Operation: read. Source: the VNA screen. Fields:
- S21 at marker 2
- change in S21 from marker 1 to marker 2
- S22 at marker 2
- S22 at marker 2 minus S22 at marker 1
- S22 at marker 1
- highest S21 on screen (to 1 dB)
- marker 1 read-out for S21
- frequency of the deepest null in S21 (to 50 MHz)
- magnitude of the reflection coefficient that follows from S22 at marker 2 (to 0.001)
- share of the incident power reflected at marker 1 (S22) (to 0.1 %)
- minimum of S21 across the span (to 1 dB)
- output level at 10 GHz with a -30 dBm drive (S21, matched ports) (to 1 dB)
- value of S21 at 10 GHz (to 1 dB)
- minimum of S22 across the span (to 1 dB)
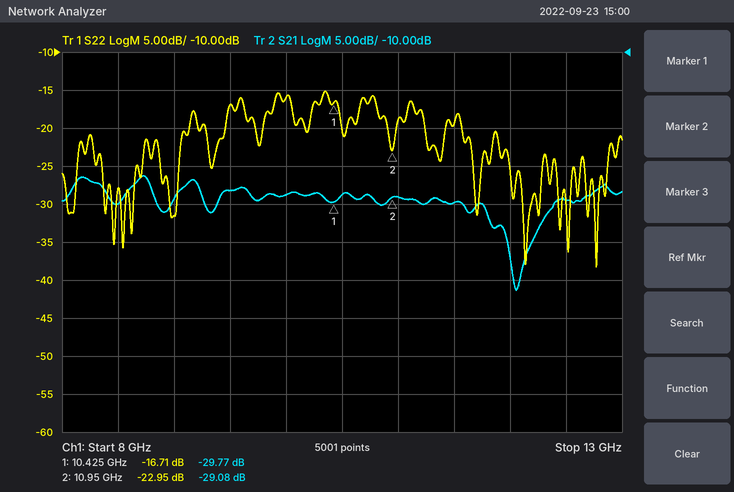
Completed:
-29.08 dB
0.69 dB
-22.95 dB
-6.24 dB
-16.71 dB
-26 dB
-29.77 dB
12.05 GHz
0.071
2.1 %
-41 dB
-59 dBm
-29 dB
-38 dB
